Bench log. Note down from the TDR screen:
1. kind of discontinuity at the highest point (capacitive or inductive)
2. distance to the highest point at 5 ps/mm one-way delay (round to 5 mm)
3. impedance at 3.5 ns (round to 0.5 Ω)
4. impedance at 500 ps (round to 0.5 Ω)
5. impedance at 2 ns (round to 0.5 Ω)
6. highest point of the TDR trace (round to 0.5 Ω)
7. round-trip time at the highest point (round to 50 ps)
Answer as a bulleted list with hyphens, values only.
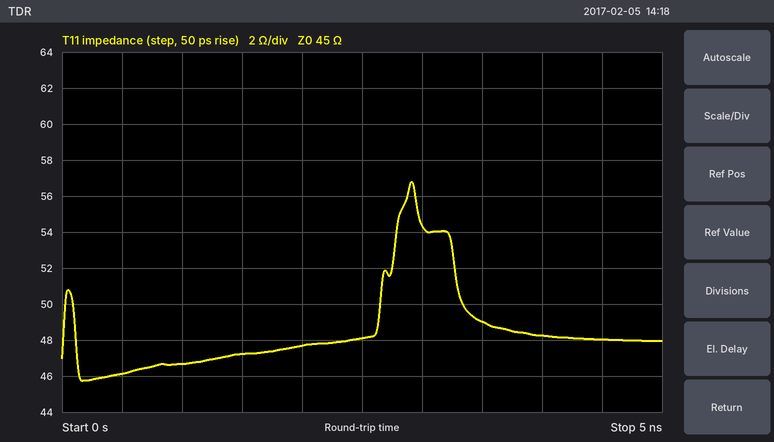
- inductive
- 290 mm
- 49.0 Ω
- 46.0 Ω
- 47.5 Ω
- 57.0 Ω
- 2.90 ns
